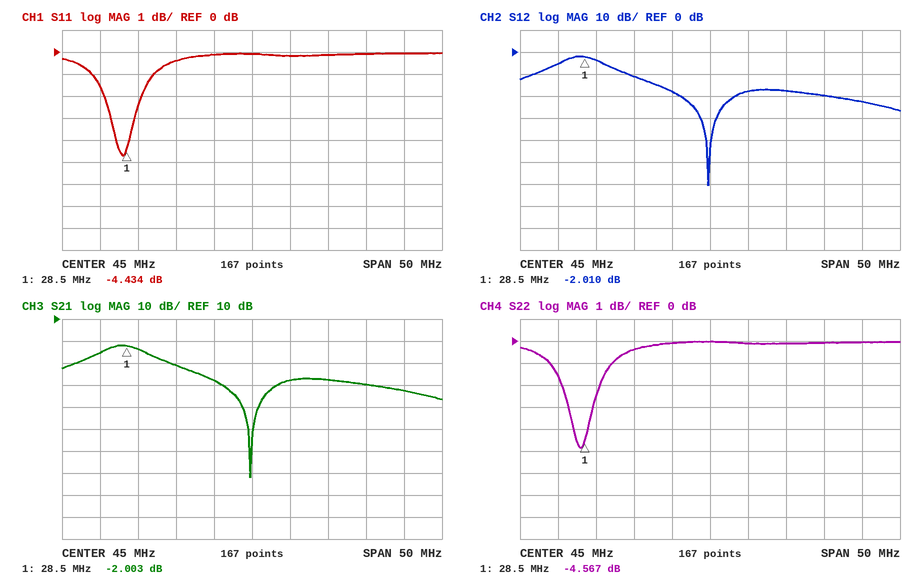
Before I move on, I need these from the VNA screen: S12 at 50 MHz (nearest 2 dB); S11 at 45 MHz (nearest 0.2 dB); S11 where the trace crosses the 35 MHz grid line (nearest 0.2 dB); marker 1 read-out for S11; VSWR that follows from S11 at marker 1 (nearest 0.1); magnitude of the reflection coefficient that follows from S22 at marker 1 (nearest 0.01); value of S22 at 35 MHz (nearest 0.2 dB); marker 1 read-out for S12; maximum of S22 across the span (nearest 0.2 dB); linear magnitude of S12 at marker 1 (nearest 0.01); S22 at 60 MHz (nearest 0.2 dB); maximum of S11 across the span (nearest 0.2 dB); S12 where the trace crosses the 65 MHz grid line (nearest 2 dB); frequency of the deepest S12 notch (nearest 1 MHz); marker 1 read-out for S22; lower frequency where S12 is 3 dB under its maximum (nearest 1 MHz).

-18 dB
0.0 dB
-0.4 dB
-4.434 dB
4.0
0.59
-0.4 dB
-2.010 dB
0.0 dB
0.79
0.0 dB
0.0 dB
-22 dB
45 MHz
-4.567 dB
25 MHz
